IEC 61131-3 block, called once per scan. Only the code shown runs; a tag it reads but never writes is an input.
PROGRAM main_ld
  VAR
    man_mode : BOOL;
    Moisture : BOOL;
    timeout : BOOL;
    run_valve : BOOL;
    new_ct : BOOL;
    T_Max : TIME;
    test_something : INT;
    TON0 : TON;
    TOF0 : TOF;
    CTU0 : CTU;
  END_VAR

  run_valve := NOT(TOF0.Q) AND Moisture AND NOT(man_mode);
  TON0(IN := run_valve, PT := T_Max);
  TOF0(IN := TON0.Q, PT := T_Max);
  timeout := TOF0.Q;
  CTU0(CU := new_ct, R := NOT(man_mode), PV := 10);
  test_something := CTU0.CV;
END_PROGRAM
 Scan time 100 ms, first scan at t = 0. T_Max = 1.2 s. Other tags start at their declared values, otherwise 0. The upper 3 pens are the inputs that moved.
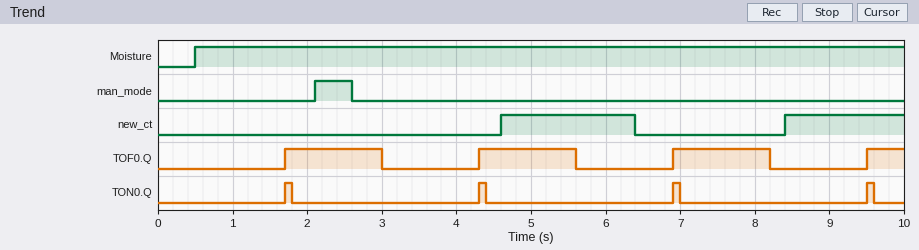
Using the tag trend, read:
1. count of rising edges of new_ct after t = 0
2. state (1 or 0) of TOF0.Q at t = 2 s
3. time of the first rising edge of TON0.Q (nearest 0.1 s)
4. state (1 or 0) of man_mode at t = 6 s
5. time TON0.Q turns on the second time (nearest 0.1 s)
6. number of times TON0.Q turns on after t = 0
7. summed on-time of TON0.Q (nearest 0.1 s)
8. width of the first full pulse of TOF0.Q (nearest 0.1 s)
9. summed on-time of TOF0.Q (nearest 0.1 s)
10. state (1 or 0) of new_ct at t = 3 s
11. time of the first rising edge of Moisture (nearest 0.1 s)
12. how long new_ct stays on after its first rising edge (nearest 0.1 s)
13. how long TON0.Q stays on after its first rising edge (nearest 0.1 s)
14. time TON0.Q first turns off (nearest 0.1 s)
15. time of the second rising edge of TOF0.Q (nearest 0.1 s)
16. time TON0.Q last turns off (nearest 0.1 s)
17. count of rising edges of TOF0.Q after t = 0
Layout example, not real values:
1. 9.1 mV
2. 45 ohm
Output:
1. 2
2. 1
3. 1.7 s
4. 0
5. 4.3 s
6. 4
7. 0.4 s
8. 1.3 s
9. 4.4 s
10. 0
11. 0.5 s
12. 1.8 s
13. 0.1 s
14. 1.8 s
15. 4.3 s
16. 9.6 s
17. 4
